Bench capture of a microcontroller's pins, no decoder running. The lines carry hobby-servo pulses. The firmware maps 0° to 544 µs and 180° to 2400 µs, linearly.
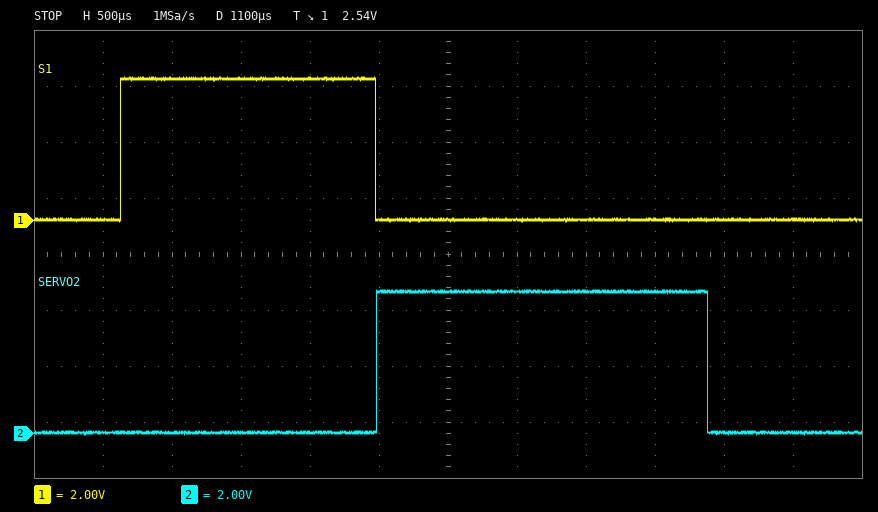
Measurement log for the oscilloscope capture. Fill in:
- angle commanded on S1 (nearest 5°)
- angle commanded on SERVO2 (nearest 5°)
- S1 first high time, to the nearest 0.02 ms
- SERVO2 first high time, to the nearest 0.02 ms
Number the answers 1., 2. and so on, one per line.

1. 125°
2. 180°
3. 1.84 ms
4. 2.40 ms
